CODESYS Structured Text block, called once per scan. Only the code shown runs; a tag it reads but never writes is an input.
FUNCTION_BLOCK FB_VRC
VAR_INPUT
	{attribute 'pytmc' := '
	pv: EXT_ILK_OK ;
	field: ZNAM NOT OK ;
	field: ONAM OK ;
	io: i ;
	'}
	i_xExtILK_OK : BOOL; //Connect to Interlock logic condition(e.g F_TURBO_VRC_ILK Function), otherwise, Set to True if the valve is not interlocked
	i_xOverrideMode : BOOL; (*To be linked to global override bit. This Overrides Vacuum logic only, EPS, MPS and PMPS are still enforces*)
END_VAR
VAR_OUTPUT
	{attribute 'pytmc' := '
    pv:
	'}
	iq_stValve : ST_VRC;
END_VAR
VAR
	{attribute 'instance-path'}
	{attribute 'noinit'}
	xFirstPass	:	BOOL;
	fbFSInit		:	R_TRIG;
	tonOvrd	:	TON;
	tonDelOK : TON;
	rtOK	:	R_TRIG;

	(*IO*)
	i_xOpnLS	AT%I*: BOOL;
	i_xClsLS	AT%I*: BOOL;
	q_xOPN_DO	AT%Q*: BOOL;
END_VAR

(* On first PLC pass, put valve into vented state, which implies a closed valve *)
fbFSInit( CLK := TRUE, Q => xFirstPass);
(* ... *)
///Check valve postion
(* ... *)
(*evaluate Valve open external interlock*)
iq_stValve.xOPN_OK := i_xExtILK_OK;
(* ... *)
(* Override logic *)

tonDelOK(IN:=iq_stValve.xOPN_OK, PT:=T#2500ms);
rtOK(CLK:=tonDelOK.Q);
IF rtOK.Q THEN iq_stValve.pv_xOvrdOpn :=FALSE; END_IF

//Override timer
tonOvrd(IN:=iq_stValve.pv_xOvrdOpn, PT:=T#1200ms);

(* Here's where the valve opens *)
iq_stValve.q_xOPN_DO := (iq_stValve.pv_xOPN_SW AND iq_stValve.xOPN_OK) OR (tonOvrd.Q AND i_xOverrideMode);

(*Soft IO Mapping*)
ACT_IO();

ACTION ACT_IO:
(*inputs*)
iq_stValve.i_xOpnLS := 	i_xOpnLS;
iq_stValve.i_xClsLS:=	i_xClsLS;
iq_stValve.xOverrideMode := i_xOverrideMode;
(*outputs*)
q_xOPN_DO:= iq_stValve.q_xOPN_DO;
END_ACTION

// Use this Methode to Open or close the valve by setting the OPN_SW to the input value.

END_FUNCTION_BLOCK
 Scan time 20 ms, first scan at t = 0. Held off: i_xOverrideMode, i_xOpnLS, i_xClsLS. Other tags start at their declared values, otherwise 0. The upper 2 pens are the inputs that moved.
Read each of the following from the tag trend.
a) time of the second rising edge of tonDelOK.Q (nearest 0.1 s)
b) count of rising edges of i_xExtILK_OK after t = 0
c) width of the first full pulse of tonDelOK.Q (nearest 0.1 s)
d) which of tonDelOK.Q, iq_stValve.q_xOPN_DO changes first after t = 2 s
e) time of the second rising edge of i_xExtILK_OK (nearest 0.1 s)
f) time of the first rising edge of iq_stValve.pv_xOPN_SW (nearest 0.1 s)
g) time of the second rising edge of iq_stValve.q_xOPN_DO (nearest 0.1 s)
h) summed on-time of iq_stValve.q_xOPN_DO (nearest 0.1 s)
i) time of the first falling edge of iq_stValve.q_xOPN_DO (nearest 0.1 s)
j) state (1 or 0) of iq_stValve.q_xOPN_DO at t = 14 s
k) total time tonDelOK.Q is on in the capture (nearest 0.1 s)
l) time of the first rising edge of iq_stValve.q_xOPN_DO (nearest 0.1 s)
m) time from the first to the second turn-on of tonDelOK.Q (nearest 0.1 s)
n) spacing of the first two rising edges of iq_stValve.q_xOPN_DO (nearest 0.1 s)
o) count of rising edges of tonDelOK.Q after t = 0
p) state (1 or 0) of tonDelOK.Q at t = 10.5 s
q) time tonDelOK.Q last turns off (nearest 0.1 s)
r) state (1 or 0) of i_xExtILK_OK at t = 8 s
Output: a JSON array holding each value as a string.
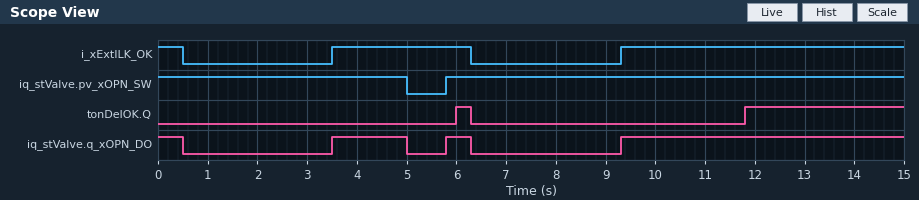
["11.8 s", "2", "0.3 s", "iq_stValve.q_xOPN_DO", "9.3 s", "5.8 s", "5.8 s", "8.2 s", "0.5 s", "1", "3.5 s", "3.5 s", "5.8 s", "2.3 s", "2", "0", "6.3 s", "0"]
